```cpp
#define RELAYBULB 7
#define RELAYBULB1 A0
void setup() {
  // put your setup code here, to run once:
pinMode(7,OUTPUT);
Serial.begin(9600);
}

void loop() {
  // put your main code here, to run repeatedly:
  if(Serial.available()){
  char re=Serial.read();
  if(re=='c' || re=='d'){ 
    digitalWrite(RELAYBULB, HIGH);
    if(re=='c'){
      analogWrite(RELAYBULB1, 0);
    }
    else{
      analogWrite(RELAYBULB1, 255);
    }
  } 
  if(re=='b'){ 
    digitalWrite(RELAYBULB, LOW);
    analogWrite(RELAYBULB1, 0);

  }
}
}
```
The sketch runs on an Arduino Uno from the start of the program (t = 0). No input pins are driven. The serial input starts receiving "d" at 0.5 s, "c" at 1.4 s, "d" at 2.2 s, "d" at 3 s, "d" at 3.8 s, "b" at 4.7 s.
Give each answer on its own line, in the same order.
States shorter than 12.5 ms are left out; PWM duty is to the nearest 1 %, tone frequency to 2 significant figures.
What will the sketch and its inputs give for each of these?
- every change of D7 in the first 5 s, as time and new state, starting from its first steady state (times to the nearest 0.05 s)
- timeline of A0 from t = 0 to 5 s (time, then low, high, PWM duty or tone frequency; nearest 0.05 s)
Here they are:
0 s low; 0.5 s high; 4.7 s low
0.5 s high; 1.4 s low; 2.2 s high; 4.7 s low
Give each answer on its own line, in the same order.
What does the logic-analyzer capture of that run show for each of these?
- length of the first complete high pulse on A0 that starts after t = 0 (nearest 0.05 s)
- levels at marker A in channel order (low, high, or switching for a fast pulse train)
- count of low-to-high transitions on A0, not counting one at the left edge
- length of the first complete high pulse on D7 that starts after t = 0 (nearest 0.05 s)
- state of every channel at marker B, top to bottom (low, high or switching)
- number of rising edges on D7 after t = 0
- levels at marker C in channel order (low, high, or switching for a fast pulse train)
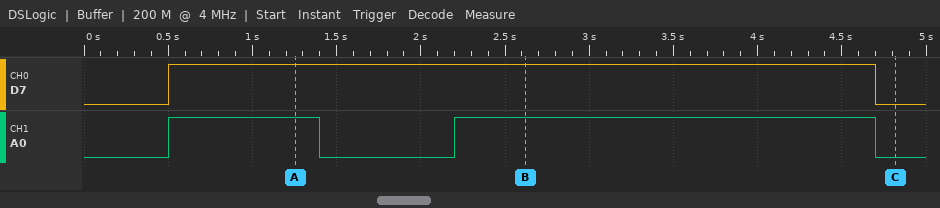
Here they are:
0.90 s
D7 high, A0 high
2
4.20 s
D7 high, A0 high
1
D7 low, A0 low
